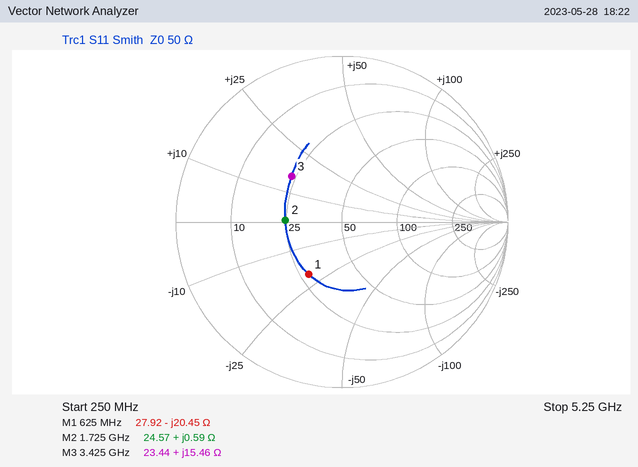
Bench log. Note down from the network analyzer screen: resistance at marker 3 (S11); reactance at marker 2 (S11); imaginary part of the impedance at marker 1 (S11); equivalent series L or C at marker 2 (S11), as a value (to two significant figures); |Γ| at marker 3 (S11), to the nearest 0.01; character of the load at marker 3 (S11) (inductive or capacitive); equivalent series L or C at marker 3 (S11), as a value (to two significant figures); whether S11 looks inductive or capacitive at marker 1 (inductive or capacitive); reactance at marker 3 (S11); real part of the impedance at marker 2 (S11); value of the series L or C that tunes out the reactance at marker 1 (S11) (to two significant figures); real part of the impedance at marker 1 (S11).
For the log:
23.44 Ω
+0.59 Ω
-20.45 Ω
54 pH
0.41
inductive
720 pH
capacitive
+15.46 Ω
24.57 Ω
5.2 nH
27.92 Ω
